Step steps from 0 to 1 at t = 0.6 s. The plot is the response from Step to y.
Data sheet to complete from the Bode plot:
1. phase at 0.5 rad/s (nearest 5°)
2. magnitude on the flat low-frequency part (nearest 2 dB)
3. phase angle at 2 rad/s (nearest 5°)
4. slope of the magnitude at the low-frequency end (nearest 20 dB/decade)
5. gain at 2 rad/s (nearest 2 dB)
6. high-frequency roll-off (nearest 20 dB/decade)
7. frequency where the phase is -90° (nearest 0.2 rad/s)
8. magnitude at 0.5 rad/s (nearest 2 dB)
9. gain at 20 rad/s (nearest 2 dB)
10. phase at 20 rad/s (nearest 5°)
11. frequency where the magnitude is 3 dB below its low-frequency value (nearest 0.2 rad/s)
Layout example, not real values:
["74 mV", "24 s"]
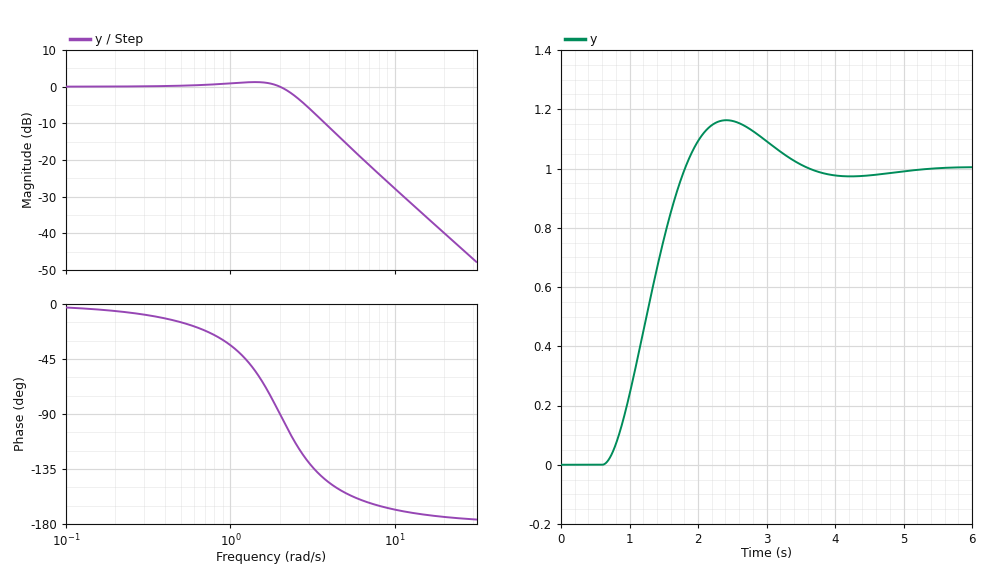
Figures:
["-15°", "0 dB", "-90°", "0 dB/decade", "0 dB", "-40 dB/decade", "2.0 rad/s", "0 dB", "-40 dB", "-175°", "2.6 rad/s"]
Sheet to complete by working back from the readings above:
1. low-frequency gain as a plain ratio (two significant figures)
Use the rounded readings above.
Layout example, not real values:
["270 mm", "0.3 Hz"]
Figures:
["1.0"]
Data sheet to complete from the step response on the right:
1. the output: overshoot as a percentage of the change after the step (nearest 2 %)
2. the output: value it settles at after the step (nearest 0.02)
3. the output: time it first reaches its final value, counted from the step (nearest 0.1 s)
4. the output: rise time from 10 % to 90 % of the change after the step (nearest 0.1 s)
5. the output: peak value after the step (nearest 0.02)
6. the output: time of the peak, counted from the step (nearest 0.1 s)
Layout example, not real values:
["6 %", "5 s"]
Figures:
["16 %", "1.00", "1.2 s", "0.8 s", "1.16", "1.8 s"]
